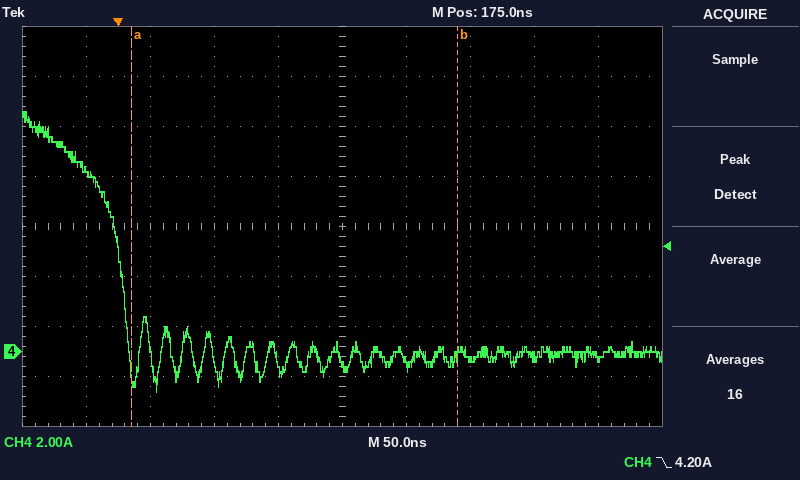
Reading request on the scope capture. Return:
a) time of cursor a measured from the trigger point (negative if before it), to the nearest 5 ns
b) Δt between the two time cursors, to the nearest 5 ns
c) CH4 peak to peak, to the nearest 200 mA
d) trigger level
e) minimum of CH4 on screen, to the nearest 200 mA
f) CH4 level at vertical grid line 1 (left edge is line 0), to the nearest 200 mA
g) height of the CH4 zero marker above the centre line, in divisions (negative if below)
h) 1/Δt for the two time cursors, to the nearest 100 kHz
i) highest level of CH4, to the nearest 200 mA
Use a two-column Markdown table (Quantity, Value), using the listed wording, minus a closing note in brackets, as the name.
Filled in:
| Quantity | Value |
|---|---|
| time of cursor a measured from the trigger point (negative if before it), to the nearest 5 ns | +10 ns |
| Δt between the two time cursors, to the nearest 5 ns | 255 ns |
| CH4 peak to peak, to the nearest 200 mA | 11.2 A |
| trigger level | 4.20 A |
| minimum of CH4 on screen, to the nearest 200 mA | -1.6 A |
| CH4 level at vertical grid line 1 (left edge is line 0), to the nearest 200 mA | 7.2 A |
| height of the CH4 zero marker above the centre line, in divisions | -2.5 div |
| 1/Δt for the two time cursors, to the nearest 100 kHz | 3.9 MHz |
| highest level of CH4, to the nearest 200 mA | 9.6 A |
